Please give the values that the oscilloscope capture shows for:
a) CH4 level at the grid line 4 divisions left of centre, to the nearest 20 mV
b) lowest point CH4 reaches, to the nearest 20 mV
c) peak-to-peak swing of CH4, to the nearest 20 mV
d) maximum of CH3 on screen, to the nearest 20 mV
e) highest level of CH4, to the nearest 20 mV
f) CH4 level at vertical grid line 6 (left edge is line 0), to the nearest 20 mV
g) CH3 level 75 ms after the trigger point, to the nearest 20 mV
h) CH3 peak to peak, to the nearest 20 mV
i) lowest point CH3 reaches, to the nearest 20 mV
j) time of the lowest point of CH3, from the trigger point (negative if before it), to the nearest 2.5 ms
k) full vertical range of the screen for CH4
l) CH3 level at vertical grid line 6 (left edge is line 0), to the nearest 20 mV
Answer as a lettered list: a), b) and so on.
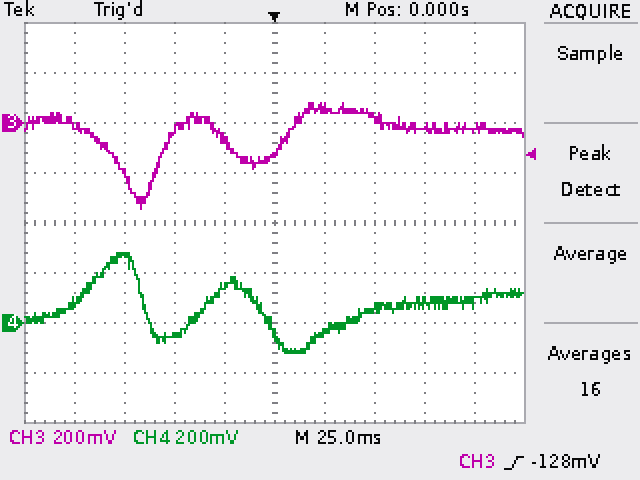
a) 80 mV
b) -120 mV
c) 400 mV
d) 80 mV
e) 280 mV
f) -40 mV
g) -20 mV
h) 420 mV
i) -340 mV
j) -67.5 ms
k) 1.6 V
l) 60 mV
